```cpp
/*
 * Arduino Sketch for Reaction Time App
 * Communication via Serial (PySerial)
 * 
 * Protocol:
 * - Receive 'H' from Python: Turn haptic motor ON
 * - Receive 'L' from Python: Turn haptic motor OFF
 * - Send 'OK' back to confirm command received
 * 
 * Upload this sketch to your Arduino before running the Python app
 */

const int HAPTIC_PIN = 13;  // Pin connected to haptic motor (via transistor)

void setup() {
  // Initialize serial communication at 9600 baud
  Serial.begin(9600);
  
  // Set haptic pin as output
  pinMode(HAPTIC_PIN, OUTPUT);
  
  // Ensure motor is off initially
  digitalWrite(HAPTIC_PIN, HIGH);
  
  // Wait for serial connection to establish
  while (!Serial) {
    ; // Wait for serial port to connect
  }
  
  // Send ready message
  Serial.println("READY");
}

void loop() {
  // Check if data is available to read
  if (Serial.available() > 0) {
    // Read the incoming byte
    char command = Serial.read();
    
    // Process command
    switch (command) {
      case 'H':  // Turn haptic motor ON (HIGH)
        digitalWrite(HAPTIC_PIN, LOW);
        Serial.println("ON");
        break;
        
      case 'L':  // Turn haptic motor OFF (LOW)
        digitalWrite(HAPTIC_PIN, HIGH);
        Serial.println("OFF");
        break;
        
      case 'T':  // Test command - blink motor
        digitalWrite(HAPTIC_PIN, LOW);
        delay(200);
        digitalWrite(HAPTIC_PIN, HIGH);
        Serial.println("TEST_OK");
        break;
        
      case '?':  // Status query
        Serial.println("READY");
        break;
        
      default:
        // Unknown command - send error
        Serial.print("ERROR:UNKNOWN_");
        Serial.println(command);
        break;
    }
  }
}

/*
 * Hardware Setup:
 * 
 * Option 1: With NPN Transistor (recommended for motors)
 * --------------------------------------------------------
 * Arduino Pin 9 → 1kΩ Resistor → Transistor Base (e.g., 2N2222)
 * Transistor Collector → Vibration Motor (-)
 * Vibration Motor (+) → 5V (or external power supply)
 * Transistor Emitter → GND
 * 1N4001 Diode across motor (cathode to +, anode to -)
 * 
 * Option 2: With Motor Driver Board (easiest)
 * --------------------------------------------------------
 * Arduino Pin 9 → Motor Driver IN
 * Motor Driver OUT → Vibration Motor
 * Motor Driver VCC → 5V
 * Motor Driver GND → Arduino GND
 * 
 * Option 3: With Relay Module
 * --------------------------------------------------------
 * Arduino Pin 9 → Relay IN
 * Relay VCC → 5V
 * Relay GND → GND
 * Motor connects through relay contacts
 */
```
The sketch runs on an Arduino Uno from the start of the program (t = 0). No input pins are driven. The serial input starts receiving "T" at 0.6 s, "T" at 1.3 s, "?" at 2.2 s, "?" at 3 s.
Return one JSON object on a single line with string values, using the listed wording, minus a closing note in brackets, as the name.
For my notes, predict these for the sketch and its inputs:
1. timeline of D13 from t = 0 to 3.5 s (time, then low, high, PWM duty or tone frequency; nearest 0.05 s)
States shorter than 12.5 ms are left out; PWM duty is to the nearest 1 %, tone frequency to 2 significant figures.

{"timeline of D13 from t = 0 to 3.5 s": "0 s high; 0.6 s low; 0.8 s high; 1.3 s low; 1.5 s high"}
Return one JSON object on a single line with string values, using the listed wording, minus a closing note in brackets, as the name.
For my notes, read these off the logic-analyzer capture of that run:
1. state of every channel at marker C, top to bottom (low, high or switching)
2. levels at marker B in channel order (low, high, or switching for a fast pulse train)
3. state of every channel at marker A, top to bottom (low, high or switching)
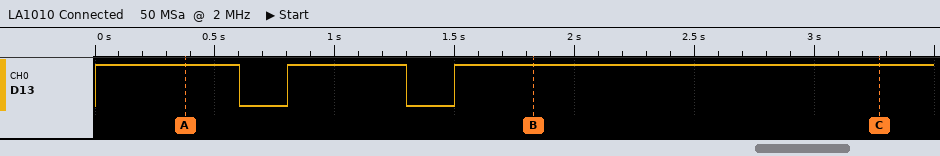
{"state of every channel at marker C, top to bottom": "D13 high", "levels at marker B in channel order": "D13 high", "state of every channel at marker A, top to bottom": "D13 high"}
